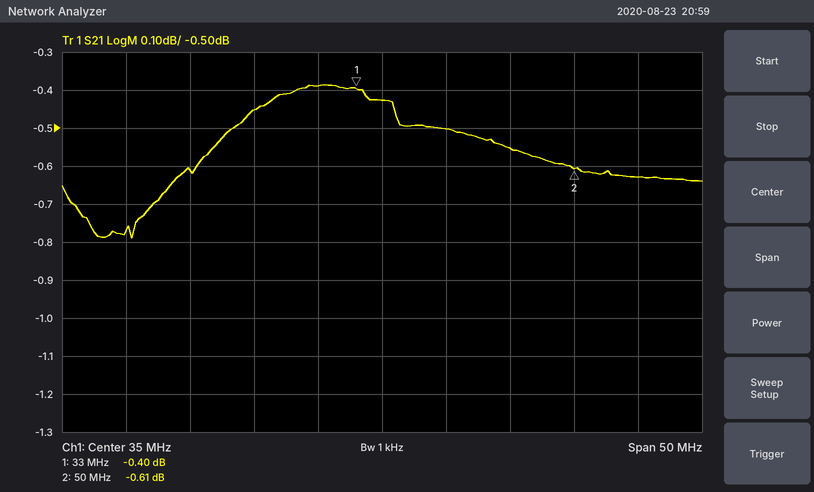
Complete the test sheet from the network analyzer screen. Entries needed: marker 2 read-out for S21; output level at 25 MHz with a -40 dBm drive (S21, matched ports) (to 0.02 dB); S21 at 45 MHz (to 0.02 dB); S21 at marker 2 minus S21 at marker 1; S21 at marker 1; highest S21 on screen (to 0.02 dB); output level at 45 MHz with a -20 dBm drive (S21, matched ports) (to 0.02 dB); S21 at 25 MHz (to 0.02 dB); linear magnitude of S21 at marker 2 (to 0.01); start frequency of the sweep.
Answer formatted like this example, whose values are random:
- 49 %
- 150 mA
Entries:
- -0.61 dB
- -40.46 dBm
- -0.56 dB
- -0.21 dB
- -0.40 dB
- -0.38 dB
- -20.56 dBm
- -0.46 dB
- 0.93
- 10 MHz
